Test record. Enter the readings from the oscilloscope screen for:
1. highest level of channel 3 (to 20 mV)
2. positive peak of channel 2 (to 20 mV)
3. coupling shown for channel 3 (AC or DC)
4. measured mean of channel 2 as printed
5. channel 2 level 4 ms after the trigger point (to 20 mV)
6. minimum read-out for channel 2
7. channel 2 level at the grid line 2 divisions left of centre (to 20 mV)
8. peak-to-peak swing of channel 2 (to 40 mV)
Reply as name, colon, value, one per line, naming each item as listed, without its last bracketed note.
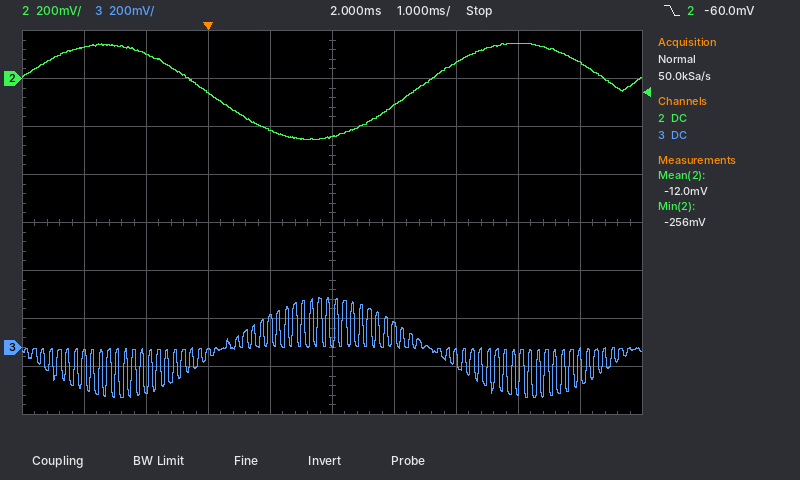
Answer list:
highest level of channel 3: 200 mV
positive peak of channel 2: 140 mV
coupling shown for channel 3: DC
measured mean of channel 2 as printed: -12.0 mV
channel 2 level 4 ms after the trigger point: 60 mV
minimum read-out for channel 2: -256 mV
channel 2 level at the grid line 2 divisions left of centre: -60 mV
peak-to-peak swing of channel 2: 400 mV
